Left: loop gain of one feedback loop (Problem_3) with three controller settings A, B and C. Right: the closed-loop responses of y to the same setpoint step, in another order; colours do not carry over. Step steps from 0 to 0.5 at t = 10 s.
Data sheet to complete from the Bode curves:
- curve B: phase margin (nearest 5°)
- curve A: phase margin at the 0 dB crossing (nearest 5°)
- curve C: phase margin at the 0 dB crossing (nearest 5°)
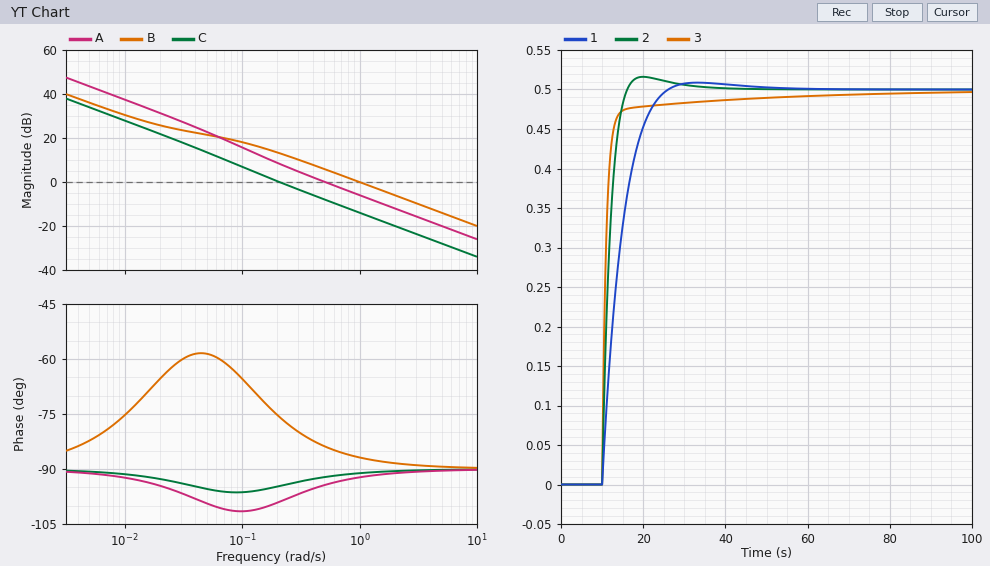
95°
85°
85°
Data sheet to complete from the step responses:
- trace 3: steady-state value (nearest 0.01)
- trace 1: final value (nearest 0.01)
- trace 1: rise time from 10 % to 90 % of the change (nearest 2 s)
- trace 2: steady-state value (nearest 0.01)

0.50
0.50
10 s
0.50
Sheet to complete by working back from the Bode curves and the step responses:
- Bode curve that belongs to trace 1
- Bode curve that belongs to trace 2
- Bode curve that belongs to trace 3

C
A
B
